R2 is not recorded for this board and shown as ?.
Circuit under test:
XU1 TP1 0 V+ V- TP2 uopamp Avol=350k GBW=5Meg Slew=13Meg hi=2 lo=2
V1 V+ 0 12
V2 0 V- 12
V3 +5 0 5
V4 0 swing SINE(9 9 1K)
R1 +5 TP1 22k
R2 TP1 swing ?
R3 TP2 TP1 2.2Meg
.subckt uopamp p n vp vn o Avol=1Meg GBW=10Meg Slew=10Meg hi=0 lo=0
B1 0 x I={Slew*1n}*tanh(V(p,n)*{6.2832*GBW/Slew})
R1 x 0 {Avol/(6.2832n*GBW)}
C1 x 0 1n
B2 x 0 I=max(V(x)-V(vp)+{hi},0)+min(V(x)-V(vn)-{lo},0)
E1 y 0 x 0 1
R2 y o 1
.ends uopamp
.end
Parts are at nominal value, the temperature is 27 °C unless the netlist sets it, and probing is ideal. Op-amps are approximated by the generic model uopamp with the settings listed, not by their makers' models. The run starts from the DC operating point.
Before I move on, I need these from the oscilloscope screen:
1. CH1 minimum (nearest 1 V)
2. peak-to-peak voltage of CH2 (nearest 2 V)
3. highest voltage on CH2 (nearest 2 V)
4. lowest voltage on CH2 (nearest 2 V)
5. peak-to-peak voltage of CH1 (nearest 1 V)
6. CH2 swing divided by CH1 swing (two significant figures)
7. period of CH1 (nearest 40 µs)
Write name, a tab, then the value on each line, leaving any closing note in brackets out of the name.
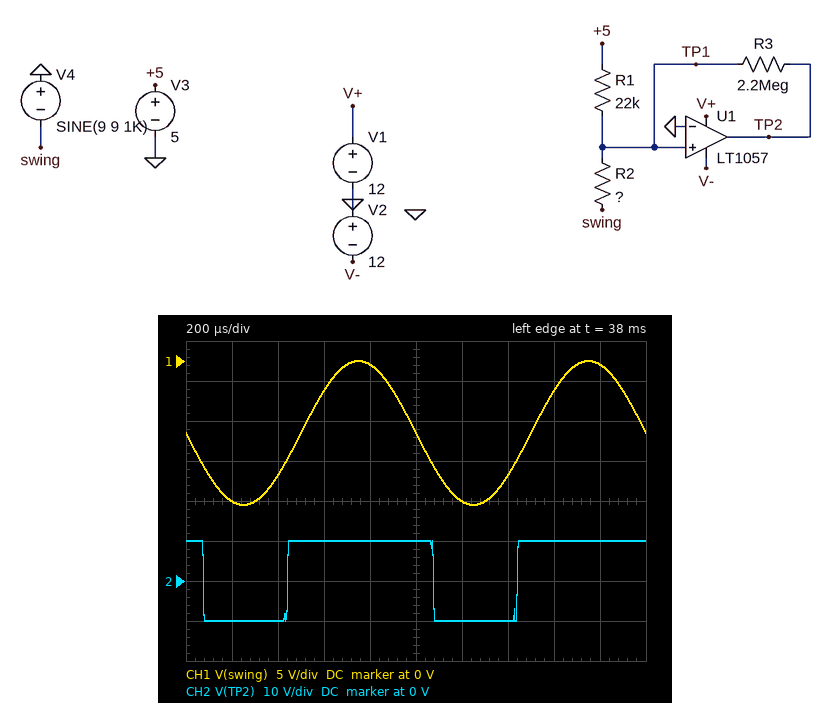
CH1 minimum	-18 V
peak-to-peak voltage of CH2	20 V
highest voltage on CH2	10 V
lowest voltage on CH2	-10 V
peak-to-peak voltage of CH1	18 V
CH2 swing divided by CH1 swing	1.1
period of CH1	1.00 ms
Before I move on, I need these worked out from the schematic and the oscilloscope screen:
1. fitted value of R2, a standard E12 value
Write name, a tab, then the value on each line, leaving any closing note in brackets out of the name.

fitted value of R2, a standard E12 value	56 kΩ
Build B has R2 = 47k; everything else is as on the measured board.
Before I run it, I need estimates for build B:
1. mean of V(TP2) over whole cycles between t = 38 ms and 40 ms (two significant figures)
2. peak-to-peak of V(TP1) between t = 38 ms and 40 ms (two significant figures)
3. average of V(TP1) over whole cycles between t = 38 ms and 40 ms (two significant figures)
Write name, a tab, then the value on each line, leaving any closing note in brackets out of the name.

mean of V(TP2) over whole cycles between t = 38 ms and 40 ms	1.2 V
peak-to-peak of V(TP1) between t = 38 ms and 40 ms	5.8 V
average of V(TP1) over whole cycles between t = 38 ms and 40 ms	540 mV
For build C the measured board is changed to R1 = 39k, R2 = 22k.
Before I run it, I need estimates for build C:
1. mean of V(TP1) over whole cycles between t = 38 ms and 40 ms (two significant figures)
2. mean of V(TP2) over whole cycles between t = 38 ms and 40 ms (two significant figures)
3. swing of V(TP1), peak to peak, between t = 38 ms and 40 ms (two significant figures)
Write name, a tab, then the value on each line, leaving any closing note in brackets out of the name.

mean of V(TP1) over whole cycles between t = 38 ms and 40 ms	-4.0 V
mean of V(TP2) over whole cycles between t = 38 ms and 40 ms	-4.8 V
swing of V(TP1), peak to peak, between t = 38 ms and 40 ms	12 V
